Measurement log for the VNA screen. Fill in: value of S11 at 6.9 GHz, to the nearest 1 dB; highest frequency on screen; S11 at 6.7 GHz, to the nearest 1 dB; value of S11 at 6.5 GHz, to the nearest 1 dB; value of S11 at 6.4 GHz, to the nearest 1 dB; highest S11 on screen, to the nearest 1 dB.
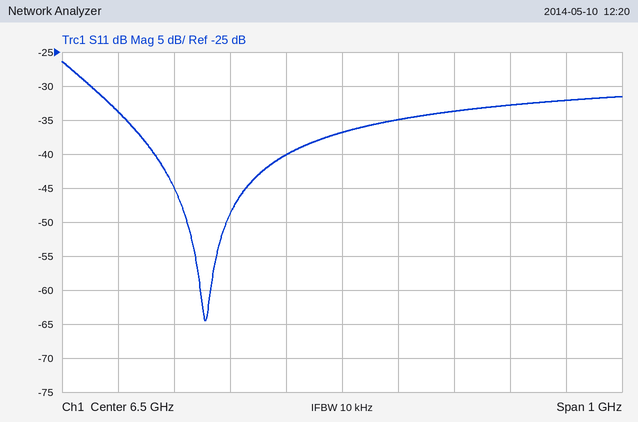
-32 dB
7 GHz
-34 dB
-37 dB
-40 dB
-26 dB
